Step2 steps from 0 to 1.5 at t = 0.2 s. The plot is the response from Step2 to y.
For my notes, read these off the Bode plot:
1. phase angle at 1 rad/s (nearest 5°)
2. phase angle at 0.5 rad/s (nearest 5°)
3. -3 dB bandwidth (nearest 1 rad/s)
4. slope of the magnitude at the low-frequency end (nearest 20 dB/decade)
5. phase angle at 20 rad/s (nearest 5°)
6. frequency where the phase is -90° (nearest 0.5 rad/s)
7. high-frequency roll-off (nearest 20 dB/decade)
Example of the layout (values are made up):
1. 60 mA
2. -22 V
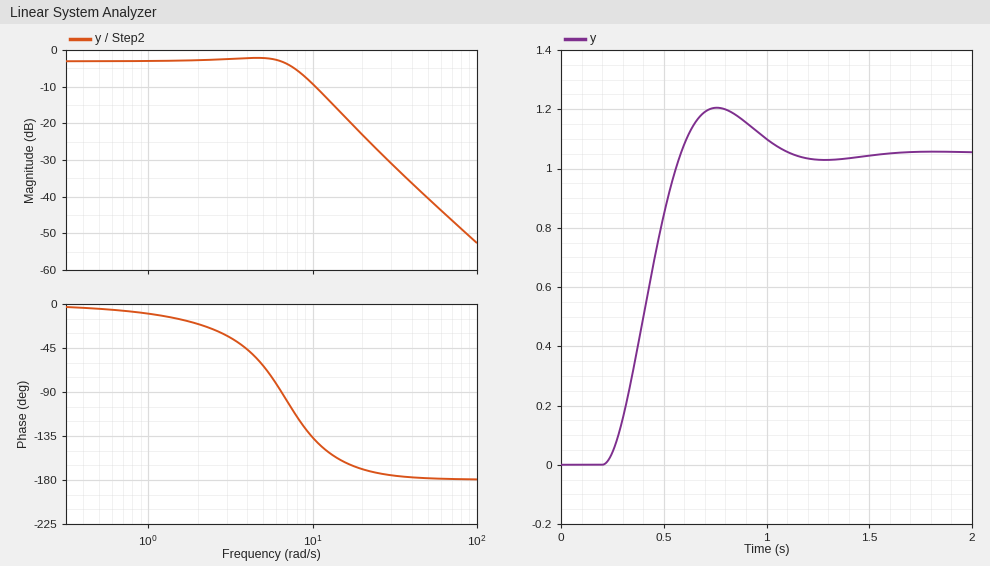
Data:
1. -10°
2. -5°
3. 8 rad/s
4. 0 dB/decade
5. -170°
6. 6.5 rad/s
7. -40 dB/decade
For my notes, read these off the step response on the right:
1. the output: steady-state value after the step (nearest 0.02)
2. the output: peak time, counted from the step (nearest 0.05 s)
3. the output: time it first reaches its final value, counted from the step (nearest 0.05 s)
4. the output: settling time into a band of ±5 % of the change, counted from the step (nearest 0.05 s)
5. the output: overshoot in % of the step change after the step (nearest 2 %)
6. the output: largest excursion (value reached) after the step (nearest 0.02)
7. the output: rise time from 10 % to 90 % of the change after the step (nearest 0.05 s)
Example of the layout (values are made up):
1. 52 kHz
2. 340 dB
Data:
1. 1.06
2. 0.55 s
3. 0.40 s
4. 0.80 s
5. 14 %
6. 1.20
7. 0.25 s
